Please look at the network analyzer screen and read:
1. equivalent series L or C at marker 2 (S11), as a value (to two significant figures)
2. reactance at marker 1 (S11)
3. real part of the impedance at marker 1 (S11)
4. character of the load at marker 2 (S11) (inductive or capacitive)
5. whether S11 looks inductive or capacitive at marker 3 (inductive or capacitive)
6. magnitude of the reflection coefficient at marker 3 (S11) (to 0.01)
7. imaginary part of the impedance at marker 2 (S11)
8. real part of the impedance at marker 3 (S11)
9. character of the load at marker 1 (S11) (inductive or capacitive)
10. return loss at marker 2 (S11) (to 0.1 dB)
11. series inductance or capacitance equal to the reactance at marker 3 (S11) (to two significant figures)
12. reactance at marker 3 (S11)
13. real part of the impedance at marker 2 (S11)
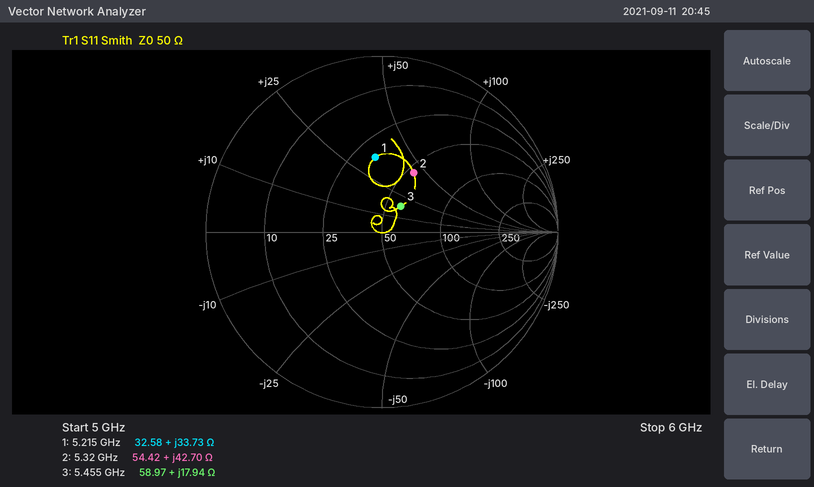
1.3 nH
+33.73 Ω
32.58 Ω
inductive
inductive
0.18
+42.70 Ω
58.97 Ω
inductive
8.4 dB
520 pH
+17.94 Ω
54.42 Ω
